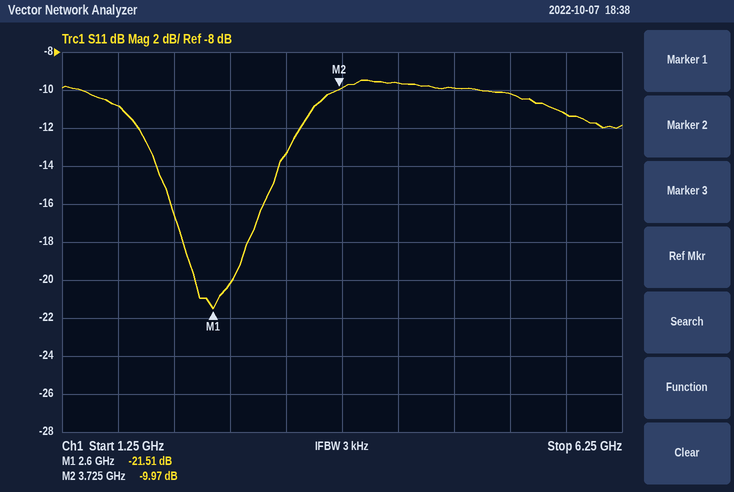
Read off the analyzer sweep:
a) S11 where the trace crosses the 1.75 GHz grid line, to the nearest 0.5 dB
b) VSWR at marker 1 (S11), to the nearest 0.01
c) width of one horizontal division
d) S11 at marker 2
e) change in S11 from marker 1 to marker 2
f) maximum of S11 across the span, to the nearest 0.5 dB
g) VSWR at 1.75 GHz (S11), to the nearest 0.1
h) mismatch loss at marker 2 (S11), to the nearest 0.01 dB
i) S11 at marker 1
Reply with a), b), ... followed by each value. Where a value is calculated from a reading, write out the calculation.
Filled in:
a) -11.0 dB
b) (1 + 0.0840)/(1 − 0.0840) ≈ 1.18
c) 500 MHz
d) -9.97 dB
e) -9.97 − (-21.51) = 11.54 dB
f) -9.5 dB
g) |Γ| = 10^(-11/20) = 0.2818; VSWR = (1 + 0.2818)/(1 − 0.2818) ≈ 1.8
h) −10 log10(1 − 10^(-9.97/10)) ≈ 0.46 dB
i) -21.51 dB
